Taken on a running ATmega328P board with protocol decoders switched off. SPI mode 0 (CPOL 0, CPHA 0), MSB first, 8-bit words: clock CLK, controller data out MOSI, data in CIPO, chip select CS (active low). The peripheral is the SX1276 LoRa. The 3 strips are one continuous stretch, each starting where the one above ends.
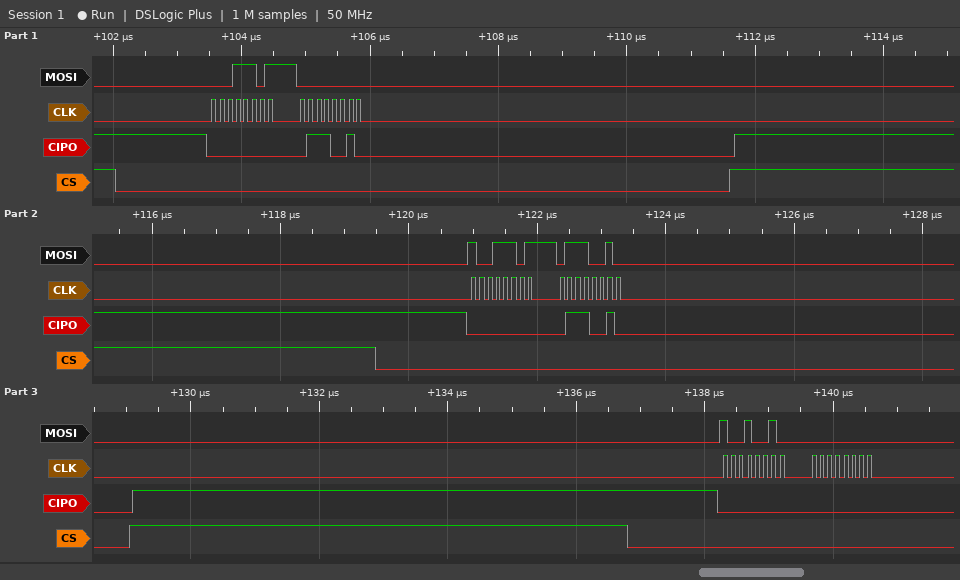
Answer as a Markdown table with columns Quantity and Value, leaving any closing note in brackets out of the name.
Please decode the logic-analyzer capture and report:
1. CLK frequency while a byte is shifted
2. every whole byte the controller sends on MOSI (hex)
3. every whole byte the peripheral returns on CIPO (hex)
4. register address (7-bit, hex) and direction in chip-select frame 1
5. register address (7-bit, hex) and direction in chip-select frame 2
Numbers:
| Quantity | Value |
|---|---|
| CLK frequency while a byte is shifted | 8 MHz |
| every whole byte the controller sends on MOSI | 0x1D 0x00 0x9D 0x72 0x92 0x00 |
| every whole byte the peripheral returns on CIPO | 0x00 0x72 0x00 0x72 0x00 0x00 |
| register address (7-bit, hex) and direction in chip-select frame 1 | 0x1D read |
| register address (7-bit, hex) and direction in chip-select frame 2 | 0x1D write |
